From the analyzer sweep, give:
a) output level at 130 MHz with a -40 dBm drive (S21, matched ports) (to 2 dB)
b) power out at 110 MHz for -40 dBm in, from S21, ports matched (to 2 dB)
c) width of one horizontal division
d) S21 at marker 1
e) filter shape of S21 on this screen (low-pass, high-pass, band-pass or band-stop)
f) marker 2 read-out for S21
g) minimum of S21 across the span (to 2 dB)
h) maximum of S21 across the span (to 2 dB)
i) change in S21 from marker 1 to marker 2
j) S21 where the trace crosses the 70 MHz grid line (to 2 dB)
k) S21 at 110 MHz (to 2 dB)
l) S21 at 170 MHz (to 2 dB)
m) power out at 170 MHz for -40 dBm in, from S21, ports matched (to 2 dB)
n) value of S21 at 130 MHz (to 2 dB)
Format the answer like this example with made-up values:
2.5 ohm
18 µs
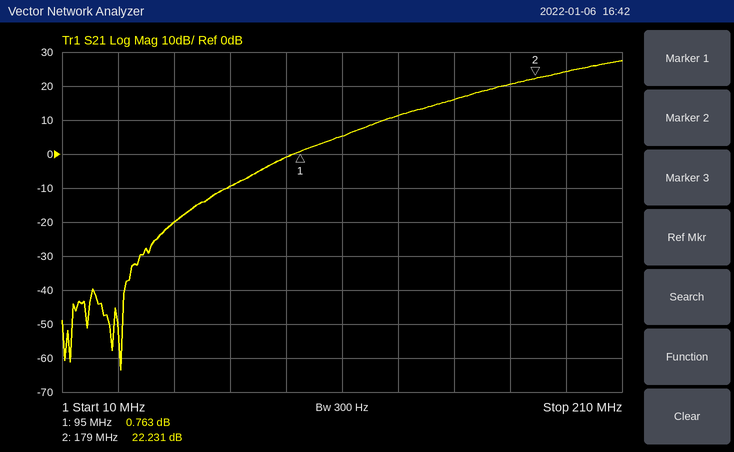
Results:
-28 dBm
-34 dBm
20 MHz
0.763 dB
high-pass
22.231 dB
-64 dB
28 dB
21.468 dB
-10 dB
6 dB
20 dB
-20 dBm
12 dB
